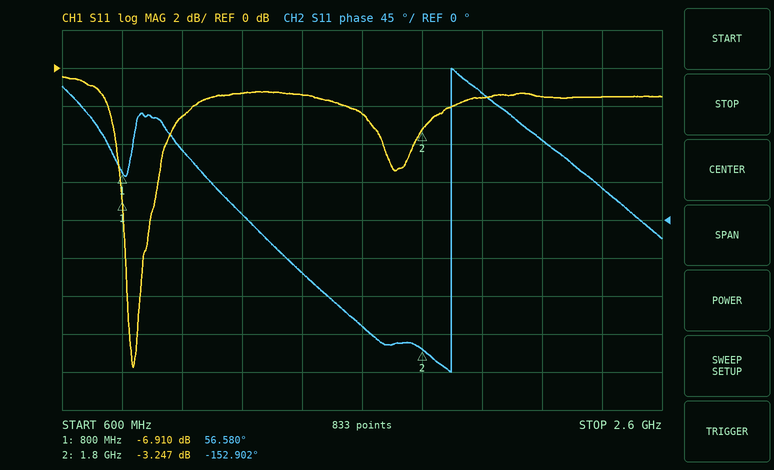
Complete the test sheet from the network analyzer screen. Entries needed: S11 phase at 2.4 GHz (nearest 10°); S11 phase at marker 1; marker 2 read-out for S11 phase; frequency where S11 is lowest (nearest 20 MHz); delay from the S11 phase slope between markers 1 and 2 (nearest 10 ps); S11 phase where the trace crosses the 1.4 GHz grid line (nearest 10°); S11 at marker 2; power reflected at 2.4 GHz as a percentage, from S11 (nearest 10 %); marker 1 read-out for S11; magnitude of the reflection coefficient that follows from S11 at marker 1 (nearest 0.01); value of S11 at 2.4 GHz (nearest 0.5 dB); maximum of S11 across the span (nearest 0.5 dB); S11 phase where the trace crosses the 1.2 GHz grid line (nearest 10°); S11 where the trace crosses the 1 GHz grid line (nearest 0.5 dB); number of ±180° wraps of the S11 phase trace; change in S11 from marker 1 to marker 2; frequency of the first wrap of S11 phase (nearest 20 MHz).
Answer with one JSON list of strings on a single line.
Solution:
["40°", "56.580°", "-152.902°", "840 MHz", "580 ps", "-60°", "-3.247 dB", "70 %", "-6.910 dB", "0.45", "-1.5 dB", "-0.5 dB", "10°", "-2.5 dB", "1", "3.663 dB", "1.90 GHz"]
